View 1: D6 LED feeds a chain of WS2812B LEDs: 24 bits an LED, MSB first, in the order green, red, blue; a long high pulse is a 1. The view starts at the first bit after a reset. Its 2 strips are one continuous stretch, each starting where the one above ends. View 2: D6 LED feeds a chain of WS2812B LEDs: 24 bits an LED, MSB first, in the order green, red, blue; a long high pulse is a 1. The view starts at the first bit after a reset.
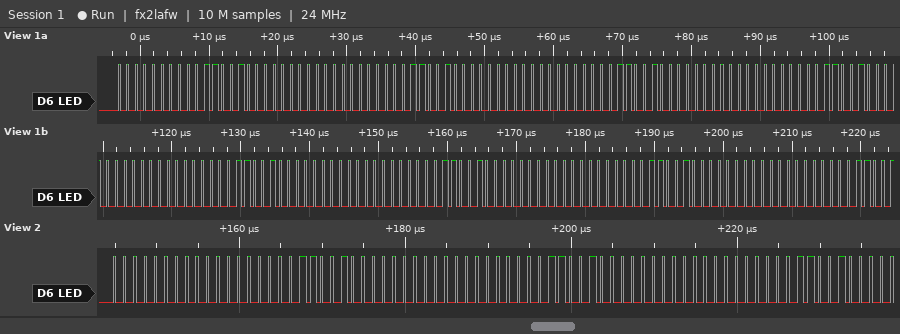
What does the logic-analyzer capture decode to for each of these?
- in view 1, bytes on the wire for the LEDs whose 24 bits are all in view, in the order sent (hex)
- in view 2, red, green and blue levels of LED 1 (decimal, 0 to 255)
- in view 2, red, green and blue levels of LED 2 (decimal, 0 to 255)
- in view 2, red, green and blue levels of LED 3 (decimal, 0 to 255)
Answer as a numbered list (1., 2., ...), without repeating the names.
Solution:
1. 00 32 00 00 32 00 00 32 00 00 32 00 00 32 00 00 32 00 00 32 00
2. 0, 0, 50
3. 0, 0, 50
4. 0, 0, 50
